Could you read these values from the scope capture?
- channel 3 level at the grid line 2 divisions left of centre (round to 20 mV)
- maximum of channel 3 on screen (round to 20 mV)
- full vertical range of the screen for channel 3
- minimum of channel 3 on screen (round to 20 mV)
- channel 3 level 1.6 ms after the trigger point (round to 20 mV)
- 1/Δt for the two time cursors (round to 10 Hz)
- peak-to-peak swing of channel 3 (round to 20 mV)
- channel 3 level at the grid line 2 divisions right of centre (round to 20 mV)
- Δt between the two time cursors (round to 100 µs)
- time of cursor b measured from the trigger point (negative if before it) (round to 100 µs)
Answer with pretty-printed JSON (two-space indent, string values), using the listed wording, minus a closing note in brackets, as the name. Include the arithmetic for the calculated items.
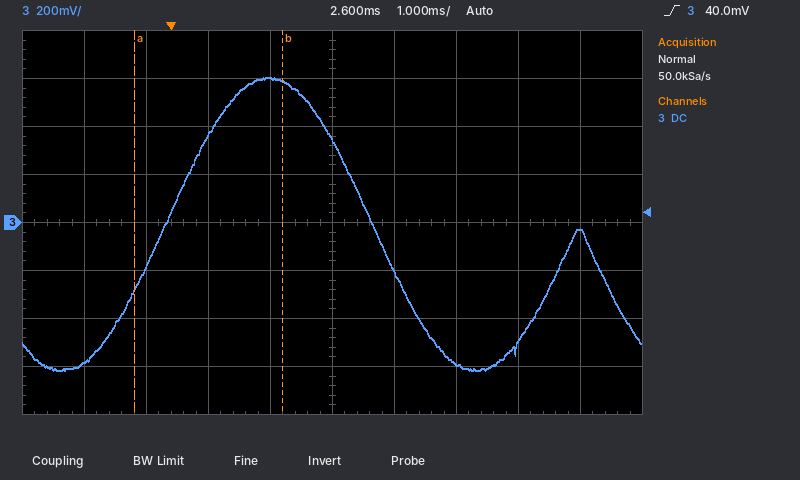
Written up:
{
  "channel 3 level at the grid line 2 divisions left of centre": "360 mV",
  "maximum of channel 3 on screen": "600 mV",
  "full vertical range of the screen for channel 3": "1.6 V",
  "minimum of channel 3 on screen": "-620 mV",
  "channel 3 level 1.6 ms after the trigger point": "600 mV",
  "1/Δt for the two time cursors": "1 / 2.4 ms ≈ 420 Hz",
  "peak-to-peak swing of channel 3": "600 mV − (-620 mV) = 1.22 V",
  "channel 3 level at the grid line 2 divisions right of centre": "-580 mV",
  "Δt between the two time cursors": "2.4 ms",
  "time of cursor b measured from the trigger point (negative if before it)": "+1.8 ms"
}
